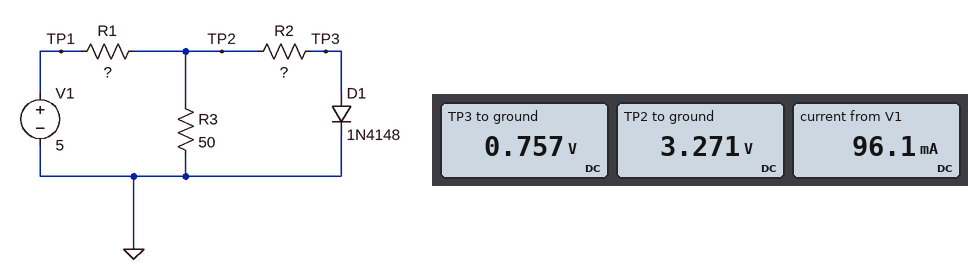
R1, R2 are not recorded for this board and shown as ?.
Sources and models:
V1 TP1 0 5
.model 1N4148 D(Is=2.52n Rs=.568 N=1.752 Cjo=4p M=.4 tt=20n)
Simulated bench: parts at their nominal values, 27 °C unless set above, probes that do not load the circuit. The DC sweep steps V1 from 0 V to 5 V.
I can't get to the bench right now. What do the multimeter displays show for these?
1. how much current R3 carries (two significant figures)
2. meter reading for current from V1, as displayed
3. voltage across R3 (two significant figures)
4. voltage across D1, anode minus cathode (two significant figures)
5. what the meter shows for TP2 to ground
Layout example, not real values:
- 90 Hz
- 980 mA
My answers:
- 65 mA
- 96.1 mA
- 3.3 V
- 760 mV
- 3.271 V
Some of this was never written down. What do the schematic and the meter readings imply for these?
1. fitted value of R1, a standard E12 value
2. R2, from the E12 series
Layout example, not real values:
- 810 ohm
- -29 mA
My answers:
- 18 Ω
- 82 Ω
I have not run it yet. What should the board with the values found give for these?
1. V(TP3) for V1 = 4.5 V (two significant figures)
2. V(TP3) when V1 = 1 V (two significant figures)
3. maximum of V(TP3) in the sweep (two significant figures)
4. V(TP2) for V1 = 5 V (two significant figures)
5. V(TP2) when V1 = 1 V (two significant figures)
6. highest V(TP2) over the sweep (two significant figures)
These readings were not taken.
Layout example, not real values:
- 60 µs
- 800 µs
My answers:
- 750 mV
- 600 mV
- 760 mV
- 3.3 V
- 720 mV
- 3.3 V
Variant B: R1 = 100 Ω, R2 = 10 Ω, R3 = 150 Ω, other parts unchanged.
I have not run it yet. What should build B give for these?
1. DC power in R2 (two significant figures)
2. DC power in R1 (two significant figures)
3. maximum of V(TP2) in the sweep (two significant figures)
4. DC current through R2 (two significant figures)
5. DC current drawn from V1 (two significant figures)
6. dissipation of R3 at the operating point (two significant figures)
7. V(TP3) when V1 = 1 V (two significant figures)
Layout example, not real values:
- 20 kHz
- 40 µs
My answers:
- 10 mW
- 150 mW
- 1.1 V
- 32 mA
- 39 mA
- 7.8 mW
- 560 mV
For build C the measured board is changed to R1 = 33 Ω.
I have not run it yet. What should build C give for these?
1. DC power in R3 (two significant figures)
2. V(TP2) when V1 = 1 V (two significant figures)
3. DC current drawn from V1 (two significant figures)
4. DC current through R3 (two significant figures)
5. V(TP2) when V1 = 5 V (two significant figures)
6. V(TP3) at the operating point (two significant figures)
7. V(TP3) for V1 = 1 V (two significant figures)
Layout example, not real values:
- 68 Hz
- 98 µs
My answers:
- 130 mW
- 590 mV
- 74 mA
- 51 mA
- 2.6 V
- 740 mV
- 550 mV
